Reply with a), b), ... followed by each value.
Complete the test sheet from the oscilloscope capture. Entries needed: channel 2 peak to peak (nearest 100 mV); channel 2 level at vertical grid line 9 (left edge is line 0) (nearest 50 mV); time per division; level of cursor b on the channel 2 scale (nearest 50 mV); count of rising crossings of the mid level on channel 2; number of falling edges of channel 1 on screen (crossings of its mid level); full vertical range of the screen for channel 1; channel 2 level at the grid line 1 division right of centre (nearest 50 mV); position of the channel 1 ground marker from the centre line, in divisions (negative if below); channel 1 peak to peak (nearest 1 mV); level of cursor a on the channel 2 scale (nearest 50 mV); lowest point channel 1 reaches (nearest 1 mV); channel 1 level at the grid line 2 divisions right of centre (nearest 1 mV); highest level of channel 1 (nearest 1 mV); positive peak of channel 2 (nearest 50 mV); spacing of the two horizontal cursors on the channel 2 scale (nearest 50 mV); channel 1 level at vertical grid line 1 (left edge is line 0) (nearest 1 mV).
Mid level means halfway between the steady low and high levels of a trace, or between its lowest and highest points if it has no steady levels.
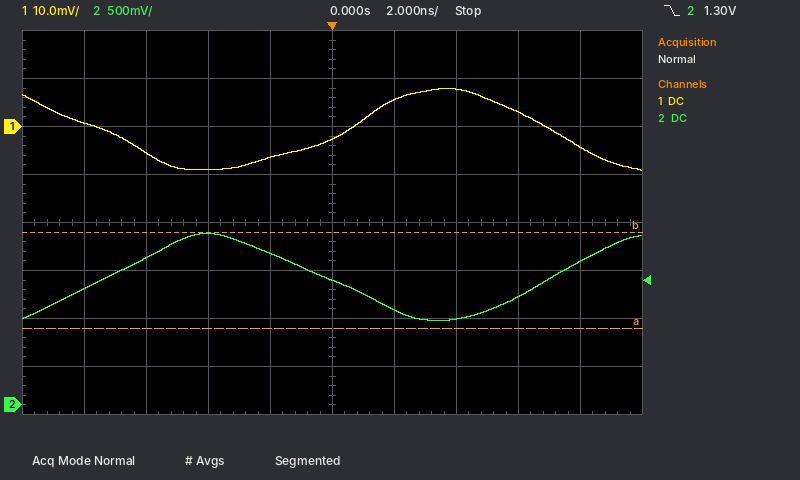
a) 900 mV
b) 1.50 V
c) 2 ns
d) 1.80 V
e) 2
f) 2
g) 80 mV
h) 1.00 V
i) +2.0 div
j) 17 mV
k) 800 mV
l) -9 mV
m) 8 mV
n) 8 mV
o) 1.80 V
p) 1.00 V
q) 1 mV
